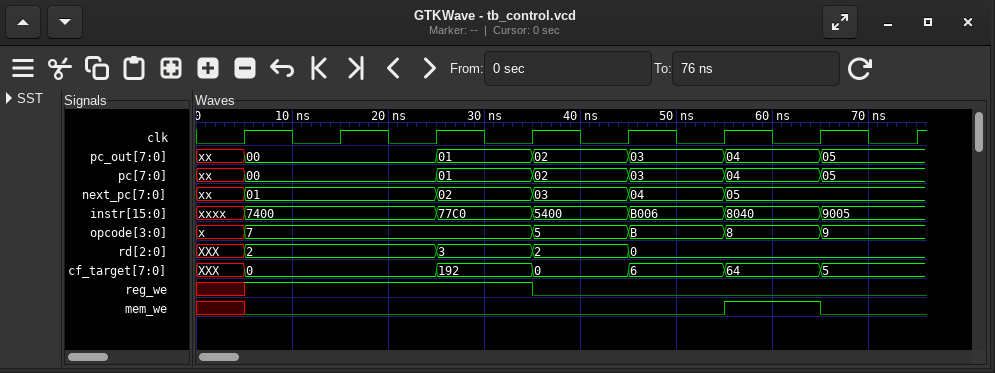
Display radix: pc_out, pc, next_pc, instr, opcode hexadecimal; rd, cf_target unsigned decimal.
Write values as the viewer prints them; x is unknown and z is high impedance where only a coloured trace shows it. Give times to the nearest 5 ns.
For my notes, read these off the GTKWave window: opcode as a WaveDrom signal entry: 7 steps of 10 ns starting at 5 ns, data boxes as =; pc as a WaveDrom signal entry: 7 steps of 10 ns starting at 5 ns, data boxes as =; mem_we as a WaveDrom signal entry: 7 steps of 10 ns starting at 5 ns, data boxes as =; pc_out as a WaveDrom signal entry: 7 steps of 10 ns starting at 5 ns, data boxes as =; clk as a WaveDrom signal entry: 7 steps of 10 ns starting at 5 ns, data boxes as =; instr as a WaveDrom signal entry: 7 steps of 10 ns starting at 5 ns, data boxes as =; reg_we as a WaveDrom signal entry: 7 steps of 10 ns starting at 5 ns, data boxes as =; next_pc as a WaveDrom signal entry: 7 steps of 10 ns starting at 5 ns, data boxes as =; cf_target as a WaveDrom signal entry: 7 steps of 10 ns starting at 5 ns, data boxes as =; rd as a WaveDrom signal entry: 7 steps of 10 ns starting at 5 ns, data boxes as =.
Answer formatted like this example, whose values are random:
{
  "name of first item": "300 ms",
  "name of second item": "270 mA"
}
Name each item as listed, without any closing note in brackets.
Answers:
{
  "opcode as a WaveDrom signal entry: 7 steps of 10 ns starting at 5 ns, data boxes as =": "{name: 'opcode', wave: '=..====', data: '7 5 B 8 9'}",
  "pc as a WaveDrom signal entry: 7 steps of 10 ns starting at 5 ns, data boxes as =": "{name: 'pc', wave: '=.=====', data: '00 01 02 03 04 05'}",
  "mem_we as a WaveDrom signal entry: 7 steps of 10 ns starting at 5 ns, data boxes as =": "{name: 'mem_we', wave: '0....10'}",
  "pc_out as a WaveDrom signal entry: 7 steps of 10 ns starting at 5 ns, data boxes as =": "{name: 'pc_out', wave: '=.=====', data: '00 01 02 03 04 05'}",
  "clk as a WaveDrom signal entry: 7 steps of 10 ns starting at 5 ns, data boxes as =": "{name: 'clk', wave: 'p......'}",
  "instr as a WaveDrom signal entry: 7 steps of 10 ns starting at 5 ns, data boxes as =": "{name: 'instr', wave: '=.=====', data: '7400 77C0 5400 B006 8040 9005'}",
  "reg_we as a WaveDrom signal entry: 7 steps of 10 ns starting at 5 ns, data boxes as =": "{name: 'reg_we', wave: '1..0...'}",
  "next_pc as a WaveDrom signal entry: 7 steps of 10 ns starting at 5 ns, data boxes as =": "{name: 'next_pc', wave: '=.====.', data: '01 02 03 04 05'}",
  "cf_target as a WaveDrom signal entry: 7 steps of 10 ns starting at 5 ns, data boxes as =": "{name: 'cf_target', wave: '=.=====', data: '0 192 0 6 64 5'}",
  "rd as a WaveDrom signal entry: 7 steps of 10 ns starting at 5 ns, data boxes as =": "{name: 'rd', wave: '=.===..', data: '2 3 2 0'}"
}
